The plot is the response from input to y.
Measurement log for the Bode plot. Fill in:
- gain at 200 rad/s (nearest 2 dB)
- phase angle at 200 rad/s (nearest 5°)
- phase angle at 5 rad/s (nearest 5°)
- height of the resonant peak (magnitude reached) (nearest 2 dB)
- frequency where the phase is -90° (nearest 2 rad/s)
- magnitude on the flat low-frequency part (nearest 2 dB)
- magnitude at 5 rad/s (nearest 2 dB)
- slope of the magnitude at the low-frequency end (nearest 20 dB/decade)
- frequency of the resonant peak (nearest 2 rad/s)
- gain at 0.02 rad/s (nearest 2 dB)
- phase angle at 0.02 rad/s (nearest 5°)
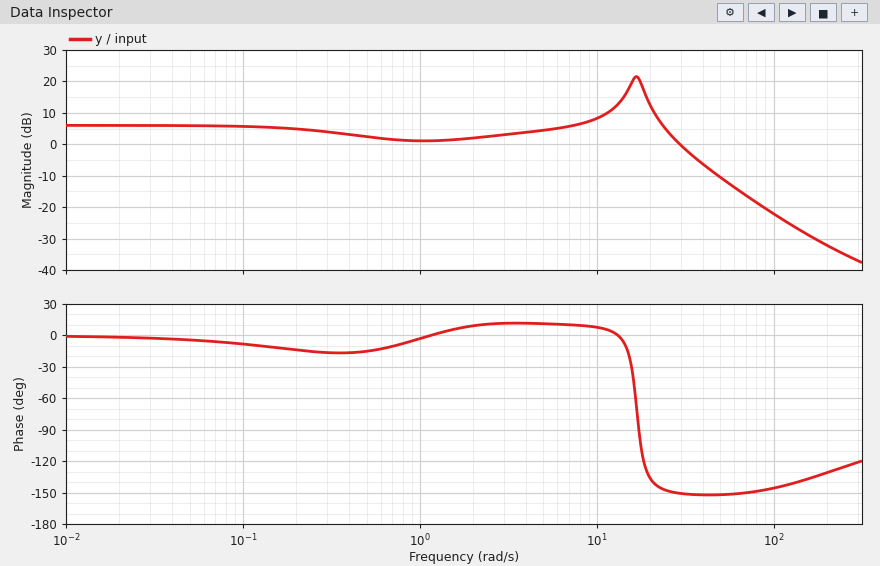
-32 dB
-130°
10°
22 dB
18 rad/s
6 dB
4 dB
0 dB/decade
16 rad/s
6 dB
0°
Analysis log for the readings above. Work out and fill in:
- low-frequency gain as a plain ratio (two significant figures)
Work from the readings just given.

2.0
